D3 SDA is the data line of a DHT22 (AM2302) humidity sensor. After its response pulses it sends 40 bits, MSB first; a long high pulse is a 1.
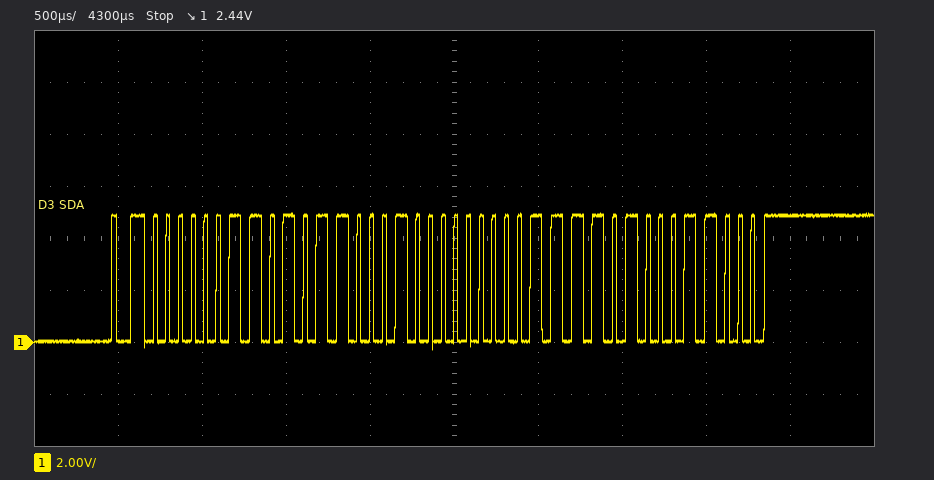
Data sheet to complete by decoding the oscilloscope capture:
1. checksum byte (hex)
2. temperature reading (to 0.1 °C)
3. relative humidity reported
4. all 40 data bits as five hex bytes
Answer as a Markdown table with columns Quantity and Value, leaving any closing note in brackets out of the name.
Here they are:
| Quantity | Value |
|---|---|
| checksum byte | 0x18 |
| temperature reading | -6.1 °C |
| relative humidity reported | 85.6 % |
| all 40 data bits as five hex bytes | 03 58 80 3D 18 |
